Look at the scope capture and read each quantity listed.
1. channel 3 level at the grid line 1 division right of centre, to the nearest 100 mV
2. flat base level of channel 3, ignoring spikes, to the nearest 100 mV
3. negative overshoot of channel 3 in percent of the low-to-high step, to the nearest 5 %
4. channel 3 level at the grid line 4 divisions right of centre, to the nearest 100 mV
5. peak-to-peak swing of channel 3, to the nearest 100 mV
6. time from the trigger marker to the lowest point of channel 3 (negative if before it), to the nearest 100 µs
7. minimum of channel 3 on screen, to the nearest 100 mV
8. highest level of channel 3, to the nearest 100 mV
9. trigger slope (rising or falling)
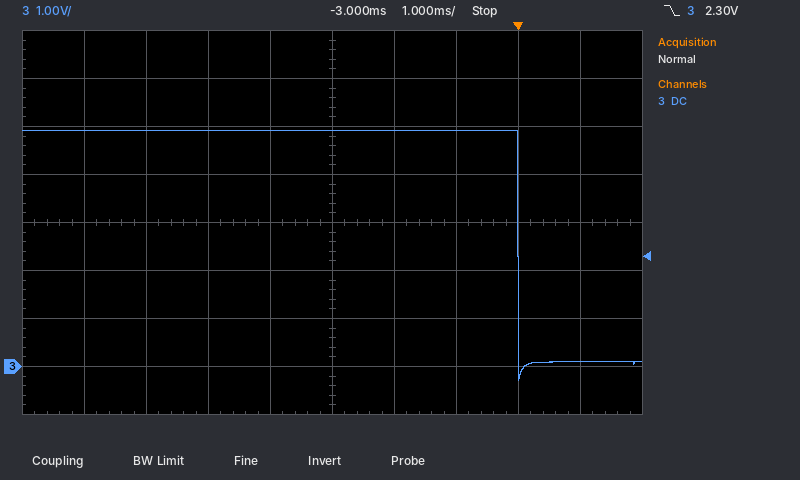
4.9 V
100 mV
10 %
100 mV
5.2 V
0.0 ms
-300 mV
4.9 V
falling
